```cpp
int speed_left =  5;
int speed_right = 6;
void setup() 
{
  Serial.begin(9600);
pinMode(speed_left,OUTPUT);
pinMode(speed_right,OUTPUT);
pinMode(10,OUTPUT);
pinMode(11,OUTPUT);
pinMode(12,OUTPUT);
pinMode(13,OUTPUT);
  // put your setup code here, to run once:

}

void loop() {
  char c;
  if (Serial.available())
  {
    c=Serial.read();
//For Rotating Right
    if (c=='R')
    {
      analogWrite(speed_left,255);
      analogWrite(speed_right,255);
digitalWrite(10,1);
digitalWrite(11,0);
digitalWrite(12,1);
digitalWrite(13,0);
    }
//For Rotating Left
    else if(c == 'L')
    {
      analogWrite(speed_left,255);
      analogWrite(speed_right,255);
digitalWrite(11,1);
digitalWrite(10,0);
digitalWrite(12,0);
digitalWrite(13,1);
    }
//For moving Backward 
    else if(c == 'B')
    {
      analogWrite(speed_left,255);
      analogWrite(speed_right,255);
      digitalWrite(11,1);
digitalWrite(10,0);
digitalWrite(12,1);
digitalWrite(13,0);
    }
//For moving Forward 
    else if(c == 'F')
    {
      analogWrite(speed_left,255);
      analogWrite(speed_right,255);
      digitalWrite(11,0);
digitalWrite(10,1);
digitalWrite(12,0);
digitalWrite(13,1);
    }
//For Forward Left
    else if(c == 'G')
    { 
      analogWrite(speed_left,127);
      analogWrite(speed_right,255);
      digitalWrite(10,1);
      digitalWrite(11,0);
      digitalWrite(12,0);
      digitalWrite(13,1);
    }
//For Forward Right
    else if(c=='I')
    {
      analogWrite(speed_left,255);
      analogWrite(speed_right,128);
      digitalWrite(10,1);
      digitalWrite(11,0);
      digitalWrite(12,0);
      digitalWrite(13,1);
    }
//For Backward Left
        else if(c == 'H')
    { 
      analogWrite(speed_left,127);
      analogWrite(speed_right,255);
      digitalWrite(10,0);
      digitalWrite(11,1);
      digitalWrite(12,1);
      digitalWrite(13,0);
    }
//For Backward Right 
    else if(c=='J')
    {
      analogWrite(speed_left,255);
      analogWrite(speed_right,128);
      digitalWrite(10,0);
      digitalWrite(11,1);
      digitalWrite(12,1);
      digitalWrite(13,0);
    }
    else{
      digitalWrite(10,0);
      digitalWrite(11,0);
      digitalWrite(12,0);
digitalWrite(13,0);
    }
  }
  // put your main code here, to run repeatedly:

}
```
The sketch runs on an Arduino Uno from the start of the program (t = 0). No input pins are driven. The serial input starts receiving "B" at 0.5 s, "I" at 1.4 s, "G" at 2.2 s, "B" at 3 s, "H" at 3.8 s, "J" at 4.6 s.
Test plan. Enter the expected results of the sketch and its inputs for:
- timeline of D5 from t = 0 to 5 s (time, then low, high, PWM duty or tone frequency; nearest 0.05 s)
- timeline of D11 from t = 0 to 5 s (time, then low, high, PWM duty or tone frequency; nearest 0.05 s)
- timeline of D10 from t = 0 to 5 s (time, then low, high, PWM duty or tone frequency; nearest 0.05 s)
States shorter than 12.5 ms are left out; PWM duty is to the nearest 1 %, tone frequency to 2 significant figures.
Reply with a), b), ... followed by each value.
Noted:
a) 0 s low; 0.5 s high; 2.2 s PWM 50 %; 3 s high; 3.8 s PWM 50 %; 4.6 s high
b) 0 s low; 0.5 s high; 1.4 s low; 3 s high
c) 0 s low; 1.4 s high; 3 s low
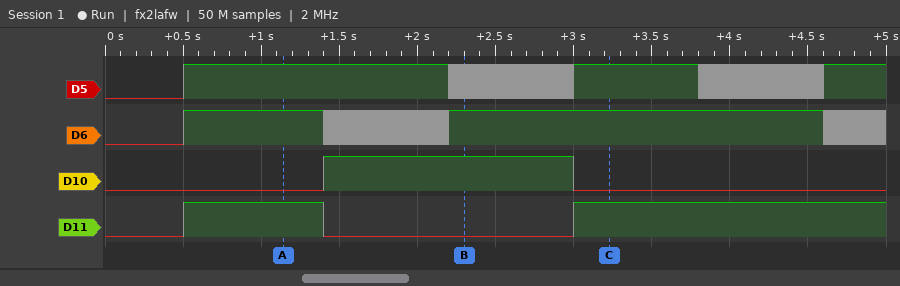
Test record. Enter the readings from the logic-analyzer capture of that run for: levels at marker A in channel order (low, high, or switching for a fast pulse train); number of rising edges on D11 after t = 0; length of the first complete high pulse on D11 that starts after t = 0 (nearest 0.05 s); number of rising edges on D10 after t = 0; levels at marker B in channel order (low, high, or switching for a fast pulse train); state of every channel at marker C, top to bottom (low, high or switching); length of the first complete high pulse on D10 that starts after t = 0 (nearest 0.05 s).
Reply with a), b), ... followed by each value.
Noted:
a) D5 high, D6 high, D10 low, D11 high
b) 2
c) 0.90 s
d) 1
e) D5 switching, D6 high, D10 high, D11 low
f) D5 high, D6 high, D10 low, D11 high
g) 1.60 s
